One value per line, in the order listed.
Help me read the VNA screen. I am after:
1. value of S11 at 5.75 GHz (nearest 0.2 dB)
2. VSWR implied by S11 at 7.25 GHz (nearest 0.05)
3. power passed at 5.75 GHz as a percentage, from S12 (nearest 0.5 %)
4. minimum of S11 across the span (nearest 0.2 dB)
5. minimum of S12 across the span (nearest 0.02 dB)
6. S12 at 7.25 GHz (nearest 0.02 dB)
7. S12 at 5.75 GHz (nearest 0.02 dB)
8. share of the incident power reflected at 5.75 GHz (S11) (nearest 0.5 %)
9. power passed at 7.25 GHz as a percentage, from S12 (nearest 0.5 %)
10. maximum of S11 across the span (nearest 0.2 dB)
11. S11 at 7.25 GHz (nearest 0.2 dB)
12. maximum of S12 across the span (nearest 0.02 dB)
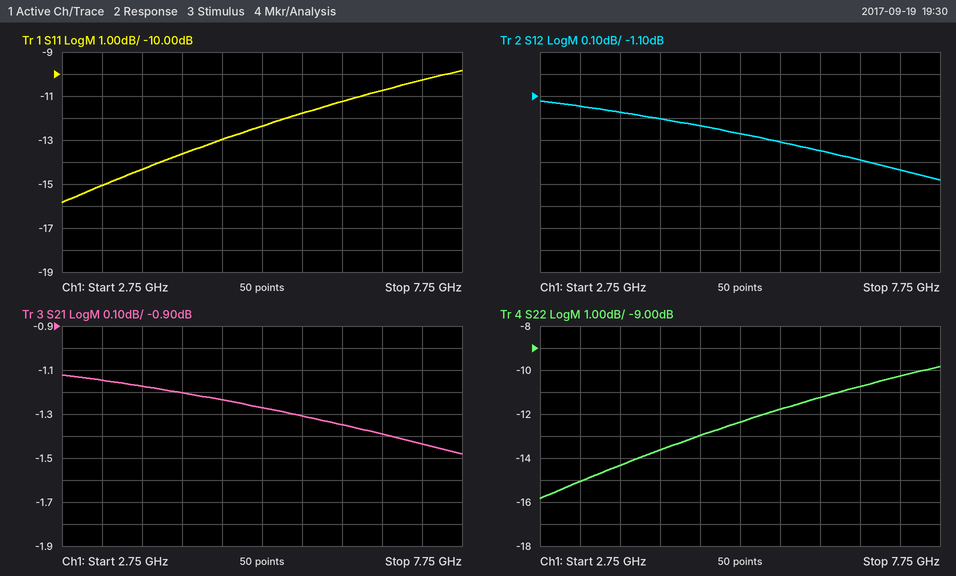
-11.8 dB
1.90
74.0 %
-15.8 dB
-1.48 dB
-1.44 dB
-1.30 dB
6.5 %
72.0 %
-9.8 dB
-10.2 dB
-1.12 dB
